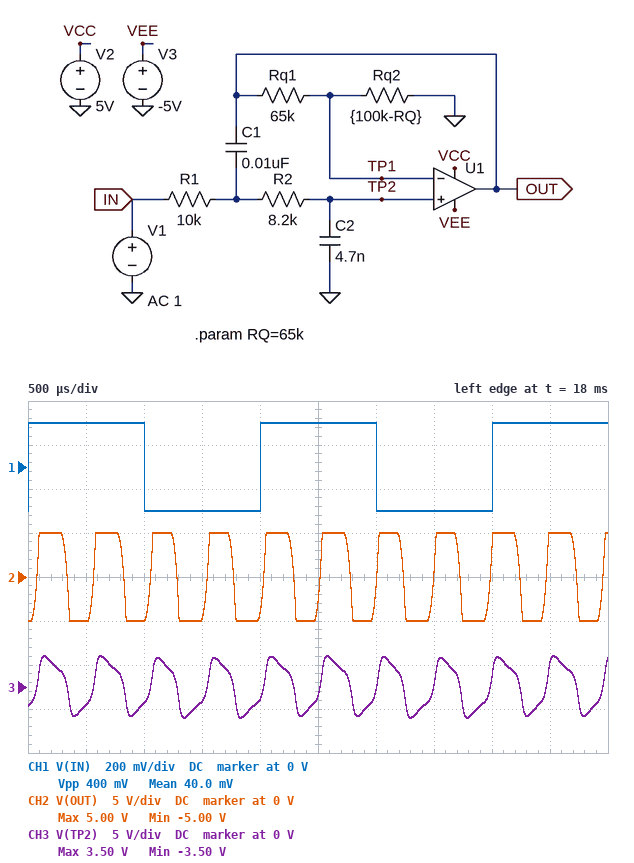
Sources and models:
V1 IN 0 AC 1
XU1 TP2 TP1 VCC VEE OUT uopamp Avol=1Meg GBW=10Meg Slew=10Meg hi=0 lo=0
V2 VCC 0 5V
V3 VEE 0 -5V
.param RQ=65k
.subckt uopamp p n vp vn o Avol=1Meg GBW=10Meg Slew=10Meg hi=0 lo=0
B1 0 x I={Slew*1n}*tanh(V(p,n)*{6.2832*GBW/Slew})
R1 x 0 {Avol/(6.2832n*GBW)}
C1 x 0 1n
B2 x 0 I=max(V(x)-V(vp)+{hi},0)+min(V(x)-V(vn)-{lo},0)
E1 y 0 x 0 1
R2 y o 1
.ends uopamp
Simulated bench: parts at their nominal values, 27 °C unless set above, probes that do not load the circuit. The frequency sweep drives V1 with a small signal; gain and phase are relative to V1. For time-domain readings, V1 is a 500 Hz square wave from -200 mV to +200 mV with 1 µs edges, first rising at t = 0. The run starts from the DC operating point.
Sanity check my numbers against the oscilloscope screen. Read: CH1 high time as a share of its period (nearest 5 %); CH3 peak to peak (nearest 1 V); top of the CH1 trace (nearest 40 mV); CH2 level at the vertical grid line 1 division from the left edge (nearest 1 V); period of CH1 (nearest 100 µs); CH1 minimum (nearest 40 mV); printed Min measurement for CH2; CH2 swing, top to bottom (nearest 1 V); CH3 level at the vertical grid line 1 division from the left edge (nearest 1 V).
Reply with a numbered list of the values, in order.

1. 50 %
2. 7 V
3. 200 mV
4. -5 V
5. 2.0 ms
6. -200 mV
7. -5.00 V
8. 10 V
9. -2 V
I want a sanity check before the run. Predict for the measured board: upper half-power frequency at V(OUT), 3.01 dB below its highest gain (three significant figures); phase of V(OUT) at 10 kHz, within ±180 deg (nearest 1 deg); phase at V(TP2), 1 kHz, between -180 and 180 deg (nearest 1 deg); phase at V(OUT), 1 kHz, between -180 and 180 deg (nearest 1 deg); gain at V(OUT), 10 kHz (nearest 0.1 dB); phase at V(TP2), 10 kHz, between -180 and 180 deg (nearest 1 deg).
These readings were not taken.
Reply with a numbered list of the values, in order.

1. 2.21 kHz
2. 156 deg
3. 37 deg
4. 37 deg
5. -14.7 dB
6. 156 deg
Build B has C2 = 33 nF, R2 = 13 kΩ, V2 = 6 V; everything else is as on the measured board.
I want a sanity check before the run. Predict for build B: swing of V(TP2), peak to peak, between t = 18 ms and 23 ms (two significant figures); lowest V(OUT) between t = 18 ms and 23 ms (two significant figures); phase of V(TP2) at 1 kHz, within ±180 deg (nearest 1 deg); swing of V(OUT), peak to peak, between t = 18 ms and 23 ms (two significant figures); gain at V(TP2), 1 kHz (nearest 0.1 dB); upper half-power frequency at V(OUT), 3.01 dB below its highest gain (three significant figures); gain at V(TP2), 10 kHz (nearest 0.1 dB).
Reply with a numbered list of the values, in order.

1. 290 mV
2. -420 mV
3. -101 deg
4. 830 mV
5. -11.3 dB
6. 318 Hz
7. -44.7 dB
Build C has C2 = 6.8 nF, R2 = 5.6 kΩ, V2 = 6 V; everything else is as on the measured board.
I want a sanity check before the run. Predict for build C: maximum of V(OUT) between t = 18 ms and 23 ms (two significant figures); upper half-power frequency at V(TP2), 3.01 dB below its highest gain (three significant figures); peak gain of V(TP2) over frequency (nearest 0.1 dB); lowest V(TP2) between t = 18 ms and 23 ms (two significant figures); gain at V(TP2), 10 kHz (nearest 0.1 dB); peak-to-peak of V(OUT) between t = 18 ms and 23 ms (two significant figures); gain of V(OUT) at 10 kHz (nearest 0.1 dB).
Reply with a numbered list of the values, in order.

1. 6.0 V
2. 2.77 kHz
3. 0.1 dB
4. -3.3 V
5. -23.5 dB
6. 11 V
7. -14.4 dB
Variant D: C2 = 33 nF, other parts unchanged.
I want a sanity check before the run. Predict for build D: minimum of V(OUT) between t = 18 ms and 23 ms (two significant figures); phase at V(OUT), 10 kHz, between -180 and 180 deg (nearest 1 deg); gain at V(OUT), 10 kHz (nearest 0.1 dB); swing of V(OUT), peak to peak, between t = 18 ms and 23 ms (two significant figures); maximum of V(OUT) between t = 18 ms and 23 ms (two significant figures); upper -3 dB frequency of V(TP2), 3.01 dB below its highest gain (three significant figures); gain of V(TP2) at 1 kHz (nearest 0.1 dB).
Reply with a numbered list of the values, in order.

1. -500 mV
2. -166 deg
3. -31.6 dB
4. 1.0 V
5. 500 mV
6. 452 Hz
7. -8.3 dB
